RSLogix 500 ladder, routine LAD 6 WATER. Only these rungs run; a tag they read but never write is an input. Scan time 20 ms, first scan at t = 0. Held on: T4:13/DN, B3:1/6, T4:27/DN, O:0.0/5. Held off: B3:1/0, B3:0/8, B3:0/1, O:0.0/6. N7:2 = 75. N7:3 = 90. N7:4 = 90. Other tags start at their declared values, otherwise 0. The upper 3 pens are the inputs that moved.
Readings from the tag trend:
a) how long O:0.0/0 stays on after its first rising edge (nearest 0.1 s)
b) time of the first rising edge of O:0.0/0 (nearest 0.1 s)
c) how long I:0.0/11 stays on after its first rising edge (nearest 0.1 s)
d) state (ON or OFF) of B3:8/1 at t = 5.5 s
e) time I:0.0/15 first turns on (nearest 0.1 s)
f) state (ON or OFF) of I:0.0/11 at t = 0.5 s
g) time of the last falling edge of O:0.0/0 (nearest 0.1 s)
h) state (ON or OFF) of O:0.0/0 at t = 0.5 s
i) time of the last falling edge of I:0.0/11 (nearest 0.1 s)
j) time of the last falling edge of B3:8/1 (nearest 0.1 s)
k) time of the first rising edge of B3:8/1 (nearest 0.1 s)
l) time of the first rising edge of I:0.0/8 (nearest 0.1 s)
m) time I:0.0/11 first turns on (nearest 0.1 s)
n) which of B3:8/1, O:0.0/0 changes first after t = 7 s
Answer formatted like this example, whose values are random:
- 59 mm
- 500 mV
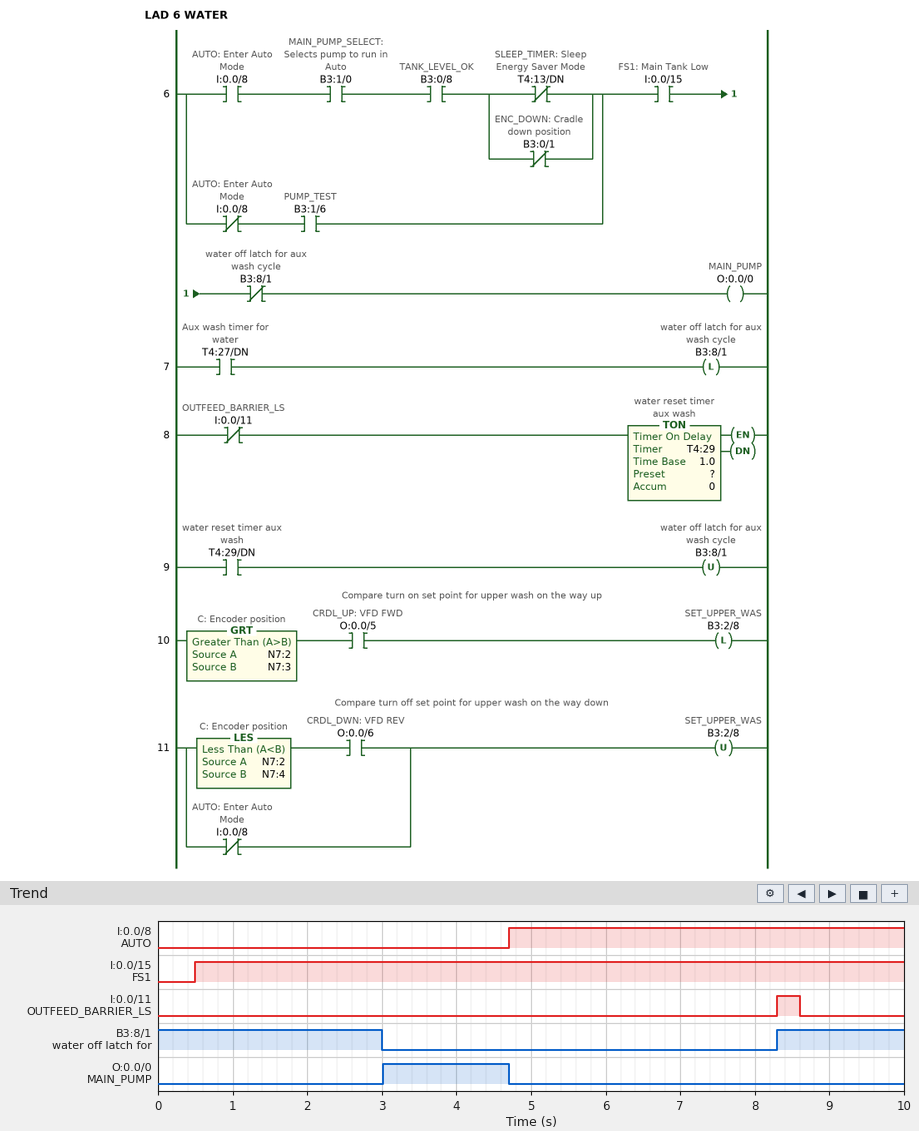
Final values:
- 1.7 s
- 3.0 s
- 0.3 s
- OFF
- 0.5 s
- OFF
- 4.7 s
- OFF
- 8.6 s
- 3.0 s
- 8.3 s
- 4.7 s
- 8.3 s
- B3:8/1
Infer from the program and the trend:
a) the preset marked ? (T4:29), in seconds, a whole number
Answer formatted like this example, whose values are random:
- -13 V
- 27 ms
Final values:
- 3 s
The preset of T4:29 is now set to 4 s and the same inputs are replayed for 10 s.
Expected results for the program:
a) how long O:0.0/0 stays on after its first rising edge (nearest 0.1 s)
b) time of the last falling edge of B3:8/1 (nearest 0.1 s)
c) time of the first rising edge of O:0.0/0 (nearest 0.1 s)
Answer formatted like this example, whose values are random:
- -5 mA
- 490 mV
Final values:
- 0.7 s
- 4.0 s
- 4.0 s
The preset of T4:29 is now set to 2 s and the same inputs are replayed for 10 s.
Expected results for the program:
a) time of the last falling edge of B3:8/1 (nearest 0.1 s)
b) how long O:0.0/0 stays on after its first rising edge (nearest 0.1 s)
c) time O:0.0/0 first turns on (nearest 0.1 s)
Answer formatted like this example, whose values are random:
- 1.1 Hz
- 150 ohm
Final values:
- 2.0 s
- 2.7 s
- 2.0 s
